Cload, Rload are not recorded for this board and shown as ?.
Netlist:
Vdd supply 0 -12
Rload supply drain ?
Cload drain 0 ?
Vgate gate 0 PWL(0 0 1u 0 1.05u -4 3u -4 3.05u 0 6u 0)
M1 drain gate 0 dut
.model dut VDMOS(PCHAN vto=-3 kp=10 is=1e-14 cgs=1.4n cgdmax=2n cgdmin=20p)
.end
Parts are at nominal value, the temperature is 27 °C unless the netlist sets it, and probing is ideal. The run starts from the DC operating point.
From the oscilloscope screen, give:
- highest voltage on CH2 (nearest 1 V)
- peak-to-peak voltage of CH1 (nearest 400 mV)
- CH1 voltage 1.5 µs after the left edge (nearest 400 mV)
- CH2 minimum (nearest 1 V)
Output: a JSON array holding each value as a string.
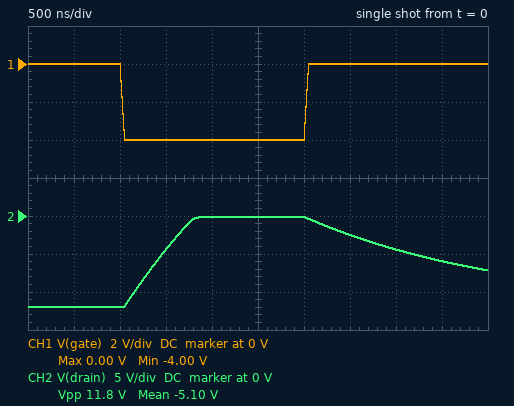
["0 V", "4.0 V", "-4.0 V", "-12 V"]
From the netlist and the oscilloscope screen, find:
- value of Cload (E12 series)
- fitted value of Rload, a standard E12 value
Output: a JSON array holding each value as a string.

["270 nF", "8.2 Ω"]
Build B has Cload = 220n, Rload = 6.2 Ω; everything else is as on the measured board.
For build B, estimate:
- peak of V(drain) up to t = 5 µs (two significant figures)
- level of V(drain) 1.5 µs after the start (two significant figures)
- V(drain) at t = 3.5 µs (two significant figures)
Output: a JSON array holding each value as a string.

["-210 mV", "-3.2 V", "-3.8 V"]
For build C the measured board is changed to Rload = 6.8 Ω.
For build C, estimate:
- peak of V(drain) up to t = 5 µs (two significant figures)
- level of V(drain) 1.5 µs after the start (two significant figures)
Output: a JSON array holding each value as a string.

["-190 mV", "-4.6 V"]
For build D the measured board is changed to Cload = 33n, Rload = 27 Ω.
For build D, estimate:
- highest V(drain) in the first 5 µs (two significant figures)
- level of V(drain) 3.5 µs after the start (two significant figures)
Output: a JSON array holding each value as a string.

["-39 mV", "-4.9 V"]
